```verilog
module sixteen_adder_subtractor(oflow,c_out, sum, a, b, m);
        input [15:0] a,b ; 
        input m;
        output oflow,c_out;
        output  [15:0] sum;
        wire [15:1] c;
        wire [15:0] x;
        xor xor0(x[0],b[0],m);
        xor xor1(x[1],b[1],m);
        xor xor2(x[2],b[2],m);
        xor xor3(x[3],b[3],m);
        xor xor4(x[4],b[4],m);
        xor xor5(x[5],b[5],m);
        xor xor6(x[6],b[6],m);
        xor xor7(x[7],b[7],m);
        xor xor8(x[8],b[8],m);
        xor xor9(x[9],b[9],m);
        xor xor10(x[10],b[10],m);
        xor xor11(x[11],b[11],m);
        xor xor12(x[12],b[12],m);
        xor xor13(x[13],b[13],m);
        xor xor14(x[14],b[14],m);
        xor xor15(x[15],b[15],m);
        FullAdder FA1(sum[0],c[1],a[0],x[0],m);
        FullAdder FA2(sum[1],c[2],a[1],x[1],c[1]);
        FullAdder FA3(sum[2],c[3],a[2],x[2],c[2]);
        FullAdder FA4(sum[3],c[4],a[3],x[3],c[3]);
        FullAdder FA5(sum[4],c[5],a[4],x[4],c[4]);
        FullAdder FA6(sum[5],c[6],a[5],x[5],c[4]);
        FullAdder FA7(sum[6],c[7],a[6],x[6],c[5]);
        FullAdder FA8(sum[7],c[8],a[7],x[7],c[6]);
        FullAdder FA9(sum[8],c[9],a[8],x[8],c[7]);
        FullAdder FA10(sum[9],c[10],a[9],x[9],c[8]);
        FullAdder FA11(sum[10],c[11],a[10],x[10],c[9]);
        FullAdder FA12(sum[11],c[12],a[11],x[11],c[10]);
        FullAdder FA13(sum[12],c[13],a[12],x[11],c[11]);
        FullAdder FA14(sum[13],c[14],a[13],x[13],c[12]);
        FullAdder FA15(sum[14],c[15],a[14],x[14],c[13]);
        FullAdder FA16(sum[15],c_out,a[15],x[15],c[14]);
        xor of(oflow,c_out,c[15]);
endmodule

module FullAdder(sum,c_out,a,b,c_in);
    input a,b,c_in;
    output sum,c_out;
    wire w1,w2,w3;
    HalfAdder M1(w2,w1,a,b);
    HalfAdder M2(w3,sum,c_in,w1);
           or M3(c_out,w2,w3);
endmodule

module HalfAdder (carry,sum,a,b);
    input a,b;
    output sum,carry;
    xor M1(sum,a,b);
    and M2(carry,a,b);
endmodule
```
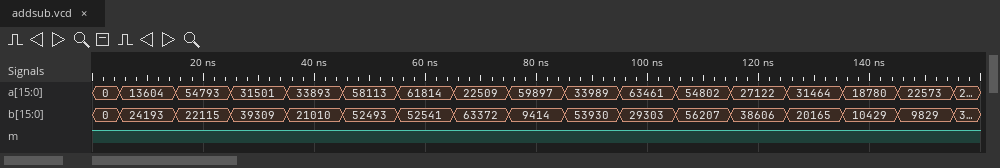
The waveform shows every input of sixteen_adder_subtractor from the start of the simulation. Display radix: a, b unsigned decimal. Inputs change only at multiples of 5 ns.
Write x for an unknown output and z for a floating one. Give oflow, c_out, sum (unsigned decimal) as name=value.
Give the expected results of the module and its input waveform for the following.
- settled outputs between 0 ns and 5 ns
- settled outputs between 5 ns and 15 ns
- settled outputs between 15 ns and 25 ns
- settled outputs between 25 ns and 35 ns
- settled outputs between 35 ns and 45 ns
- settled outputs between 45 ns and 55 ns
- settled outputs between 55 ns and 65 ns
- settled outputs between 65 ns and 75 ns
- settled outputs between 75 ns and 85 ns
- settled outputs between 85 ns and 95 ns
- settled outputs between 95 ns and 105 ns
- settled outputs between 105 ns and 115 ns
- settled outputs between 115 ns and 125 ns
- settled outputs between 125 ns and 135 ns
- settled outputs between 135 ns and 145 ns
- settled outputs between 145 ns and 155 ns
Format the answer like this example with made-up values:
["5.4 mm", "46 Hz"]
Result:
["oflow=0, c_out=1, sum=0", "oflow=1, c_out=1, sum=16803", "oflow=0, c_out=1, sum=12262", "oflow=1, c_out=0, sum=57472", "oflow=1, c_out=1, sum=28211", "oflow=1, c_out=1, sum=18932", "oflow=1, c_out=1, sum=22201", "oflow=1, c_out=0, sum=12385", "oflow=0, c_out=1, sum=40243", "oflow=0, c_out=0, sum=60571", "oflow=0, c_out=1, sum=37998", "oflow=1, c_out=0, sum=41763", "oflow=1, c_out=0, sum=46852", "oflow=1, c_out=1, sum=29731", "oflow=1, c_out=0, sum=39711", "oflow=1, c_out=0, sum=58184"]
